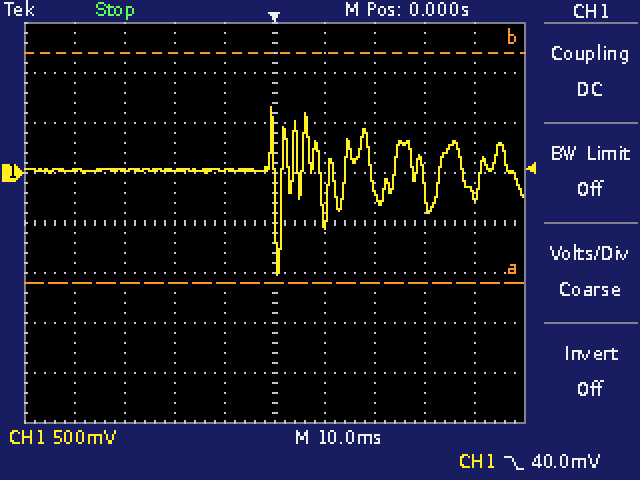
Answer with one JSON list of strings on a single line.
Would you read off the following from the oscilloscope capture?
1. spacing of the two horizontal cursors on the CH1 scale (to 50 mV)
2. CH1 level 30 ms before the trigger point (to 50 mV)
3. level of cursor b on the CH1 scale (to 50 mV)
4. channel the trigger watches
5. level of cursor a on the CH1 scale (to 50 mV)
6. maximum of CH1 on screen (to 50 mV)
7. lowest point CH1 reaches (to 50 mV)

["2.30 V", "50 mV", "1.20 V", "CH1", "-1.10 V", "650 mV", "-1.00 V"]
